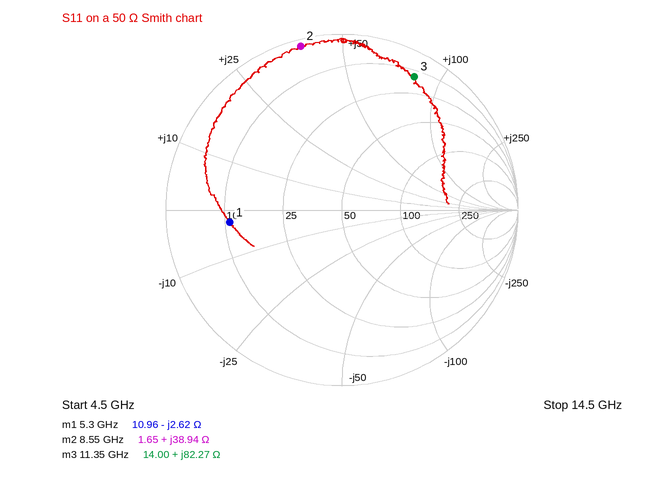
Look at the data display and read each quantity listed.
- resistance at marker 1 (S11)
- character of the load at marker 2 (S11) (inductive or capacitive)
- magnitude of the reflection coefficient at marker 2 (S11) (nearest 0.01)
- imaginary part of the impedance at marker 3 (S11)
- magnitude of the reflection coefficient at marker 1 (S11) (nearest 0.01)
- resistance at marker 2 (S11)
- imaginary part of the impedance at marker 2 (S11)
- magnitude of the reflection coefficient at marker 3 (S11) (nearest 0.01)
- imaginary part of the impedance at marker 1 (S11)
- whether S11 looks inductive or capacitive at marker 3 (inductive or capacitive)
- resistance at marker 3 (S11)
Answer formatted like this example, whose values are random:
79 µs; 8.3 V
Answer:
10.96 Ω; inductive; 0.96; +82.27 Ω; 0.64; 1.65 Ω; +38.94 Ω; 0.86; -2.62 Ω; inductive; 14.00 Ω
